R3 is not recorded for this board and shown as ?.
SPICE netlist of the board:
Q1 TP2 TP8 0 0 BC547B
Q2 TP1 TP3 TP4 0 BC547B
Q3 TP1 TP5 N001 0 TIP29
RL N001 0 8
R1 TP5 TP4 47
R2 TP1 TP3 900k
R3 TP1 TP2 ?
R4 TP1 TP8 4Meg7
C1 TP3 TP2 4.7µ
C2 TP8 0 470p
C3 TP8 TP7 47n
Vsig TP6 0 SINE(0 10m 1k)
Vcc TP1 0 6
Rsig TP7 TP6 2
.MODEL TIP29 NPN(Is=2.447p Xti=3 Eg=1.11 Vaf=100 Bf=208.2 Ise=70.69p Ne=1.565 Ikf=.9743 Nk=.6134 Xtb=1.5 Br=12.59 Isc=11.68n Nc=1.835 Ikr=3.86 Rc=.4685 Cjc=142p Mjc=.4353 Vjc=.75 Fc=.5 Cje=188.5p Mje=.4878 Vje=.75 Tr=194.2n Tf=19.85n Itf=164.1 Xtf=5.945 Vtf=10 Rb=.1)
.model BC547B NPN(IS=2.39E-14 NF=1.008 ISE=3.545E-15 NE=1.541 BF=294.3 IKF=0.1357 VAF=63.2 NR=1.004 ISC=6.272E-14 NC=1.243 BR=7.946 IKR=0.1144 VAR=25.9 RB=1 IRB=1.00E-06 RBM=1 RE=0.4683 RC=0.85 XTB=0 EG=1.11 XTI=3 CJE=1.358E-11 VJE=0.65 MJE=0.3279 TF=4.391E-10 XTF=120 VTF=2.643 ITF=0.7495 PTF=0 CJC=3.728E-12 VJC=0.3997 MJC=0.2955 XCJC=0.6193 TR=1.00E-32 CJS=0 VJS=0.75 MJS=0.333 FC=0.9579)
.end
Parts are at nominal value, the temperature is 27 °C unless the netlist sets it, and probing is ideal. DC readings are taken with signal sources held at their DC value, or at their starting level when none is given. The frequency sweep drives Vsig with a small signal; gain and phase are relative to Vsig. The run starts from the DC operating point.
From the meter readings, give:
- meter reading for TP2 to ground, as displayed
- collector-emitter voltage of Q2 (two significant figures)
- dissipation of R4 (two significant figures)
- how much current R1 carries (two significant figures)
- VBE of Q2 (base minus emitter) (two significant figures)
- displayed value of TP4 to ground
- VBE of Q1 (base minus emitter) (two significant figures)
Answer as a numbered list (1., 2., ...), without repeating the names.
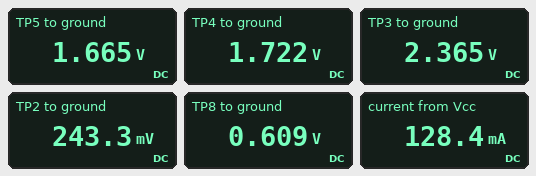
1. 243.3 mV
2. 4.3 V
3. 6.2 µW
4. 1.2 mA
5. 640 mV
6. 1.722 V
7. 610 mV
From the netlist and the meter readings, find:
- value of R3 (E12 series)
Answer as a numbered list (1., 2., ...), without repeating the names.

1. 18 kΩ
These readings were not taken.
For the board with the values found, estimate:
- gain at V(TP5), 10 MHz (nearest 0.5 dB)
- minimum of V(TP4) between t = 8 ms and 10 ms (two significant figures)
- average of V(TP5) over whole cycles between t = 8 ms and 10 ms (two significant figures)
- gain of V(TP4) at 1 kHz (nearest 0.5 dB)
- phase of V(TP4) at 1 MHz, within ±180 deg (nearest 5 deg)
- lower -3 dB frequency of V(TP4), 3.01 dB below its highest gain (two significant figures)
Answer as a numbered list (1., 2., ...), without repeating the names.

1. -1.0 dB
2. 1.6 V
3. 2.6 V
4. 44.0 dB
5. 95 deg
6. 330 Hz
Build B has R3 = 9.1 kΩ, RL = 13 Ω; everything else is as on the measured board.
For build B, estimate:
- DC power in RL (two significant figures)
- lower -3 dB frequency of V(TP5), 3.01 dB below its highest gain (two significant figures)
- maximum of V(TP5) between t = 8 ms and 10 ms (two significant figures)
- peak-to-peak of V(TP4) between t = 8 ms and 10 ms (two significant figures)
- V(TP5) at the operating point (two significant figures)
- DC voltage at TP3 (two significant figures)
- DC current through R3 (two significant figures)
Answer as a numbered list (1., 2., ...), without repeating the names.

1. 160 mW
2. 150 Hz
3. 3.0 V
4. 2.0 V
5. 2.1 V
6. 2.8 V
7. 340 µA
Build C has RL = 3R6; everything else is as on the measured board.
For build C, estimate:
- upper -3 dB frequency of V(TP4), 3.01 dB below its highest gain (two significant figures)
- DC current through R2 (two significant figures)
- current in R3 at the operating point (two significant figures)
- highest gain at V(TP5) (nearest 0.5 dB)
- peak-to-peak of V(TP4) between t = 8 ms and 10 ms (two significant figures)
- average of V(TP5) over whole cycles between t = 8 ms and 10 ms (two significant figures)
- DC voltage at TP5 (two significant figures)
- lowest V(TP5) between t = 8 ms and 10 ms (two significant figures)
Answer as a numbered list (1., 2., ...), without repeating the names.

1. 380 kHz
2. 4.6 µA
3. 320 µA
4. 43.0 dB
5. 2.2 V
6. 2.0 V
7. 1.2 V
8. 1.0 V
